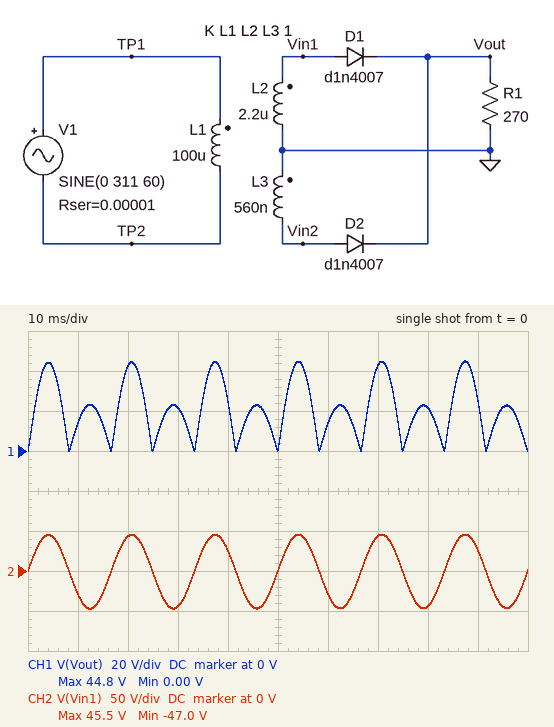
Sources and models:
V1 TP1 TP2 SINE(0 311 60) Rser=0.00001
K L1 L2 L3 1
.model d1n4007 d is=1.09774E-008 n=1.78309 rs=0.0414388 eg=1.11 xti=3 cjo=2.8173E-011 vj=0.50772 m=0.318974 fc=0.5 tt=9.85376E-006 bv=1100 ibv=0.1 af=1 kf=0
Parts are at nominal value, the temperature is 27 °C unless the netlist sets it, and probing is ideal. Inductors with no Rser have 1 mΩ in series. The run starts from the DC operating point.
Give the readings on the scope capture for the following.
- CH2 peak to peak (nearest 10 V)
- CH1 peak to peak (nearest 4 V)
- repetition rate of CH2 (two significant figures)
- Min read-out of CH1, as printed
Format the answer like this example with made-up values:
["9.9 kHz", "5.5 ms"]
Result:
["90 V", "44 V", "60 Hz", "0.00 V"]
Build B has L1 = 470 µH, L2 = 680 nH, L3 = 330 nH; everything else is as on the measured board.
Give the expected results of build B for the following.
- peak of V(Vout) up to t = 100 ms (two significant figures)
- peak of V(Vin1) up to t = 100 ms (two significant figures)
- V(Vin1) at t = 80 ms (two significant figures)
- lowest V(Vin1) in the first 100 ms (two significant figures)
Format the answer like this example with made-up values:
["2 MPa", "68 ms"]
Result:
["11 V", "12 V", "-11 V", "-12 V"]
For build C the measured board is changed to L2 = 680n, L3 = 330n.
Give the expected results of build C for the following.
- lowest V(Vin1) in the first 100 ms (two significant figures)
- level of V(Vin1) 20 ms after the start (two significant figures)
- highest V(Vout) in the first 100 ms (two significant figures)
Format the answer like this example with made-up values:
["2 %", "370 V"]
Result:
["-26 V", "24 V", "25 V"]
